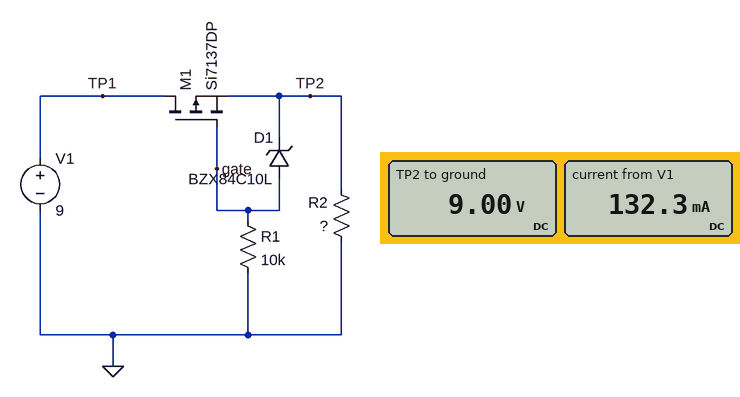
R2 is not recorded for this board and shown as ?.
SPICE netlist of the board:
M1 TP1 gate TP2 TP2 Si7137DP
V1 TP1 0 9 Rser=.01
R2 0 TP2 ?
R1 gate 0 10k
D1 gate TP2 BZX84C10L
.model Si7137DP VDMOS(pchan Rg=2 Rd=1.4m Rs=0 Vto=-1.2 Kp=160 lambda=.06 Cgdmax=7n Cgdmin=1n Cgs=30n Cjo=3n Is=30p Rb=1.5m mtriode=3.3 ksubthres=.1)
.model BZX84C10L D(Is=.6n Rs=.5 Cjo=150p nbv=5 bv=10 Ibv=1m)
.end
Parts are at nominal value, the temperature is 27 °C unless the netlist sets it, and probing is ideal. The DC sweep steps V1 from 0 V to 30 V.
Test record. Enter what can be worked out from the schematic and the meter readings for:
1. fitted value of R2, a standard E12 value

68 Ω
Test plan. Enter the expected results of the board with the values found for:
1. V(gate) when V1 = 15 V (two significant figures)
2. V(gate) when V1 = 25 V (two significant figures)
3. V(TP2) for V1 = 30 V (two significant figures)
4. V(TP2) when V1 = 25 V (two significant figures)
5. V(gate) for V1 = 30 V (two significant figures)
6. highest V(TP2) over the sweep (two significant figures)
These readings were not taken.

5.1 V
15 V
30 V
25 V
20 V
30 V
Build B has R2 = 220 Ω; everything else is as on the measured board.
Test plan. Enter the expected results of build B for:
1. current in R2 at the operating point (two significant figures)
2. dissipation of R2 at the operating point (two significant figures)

41 mA
370 mW
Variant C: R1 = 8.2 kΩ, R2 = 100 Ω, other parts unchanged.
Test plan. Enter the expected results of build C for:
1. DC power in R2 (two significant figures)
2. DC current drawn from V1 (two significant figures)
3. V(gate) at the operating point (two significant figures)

810 mW
90 mA
3.5 mV
